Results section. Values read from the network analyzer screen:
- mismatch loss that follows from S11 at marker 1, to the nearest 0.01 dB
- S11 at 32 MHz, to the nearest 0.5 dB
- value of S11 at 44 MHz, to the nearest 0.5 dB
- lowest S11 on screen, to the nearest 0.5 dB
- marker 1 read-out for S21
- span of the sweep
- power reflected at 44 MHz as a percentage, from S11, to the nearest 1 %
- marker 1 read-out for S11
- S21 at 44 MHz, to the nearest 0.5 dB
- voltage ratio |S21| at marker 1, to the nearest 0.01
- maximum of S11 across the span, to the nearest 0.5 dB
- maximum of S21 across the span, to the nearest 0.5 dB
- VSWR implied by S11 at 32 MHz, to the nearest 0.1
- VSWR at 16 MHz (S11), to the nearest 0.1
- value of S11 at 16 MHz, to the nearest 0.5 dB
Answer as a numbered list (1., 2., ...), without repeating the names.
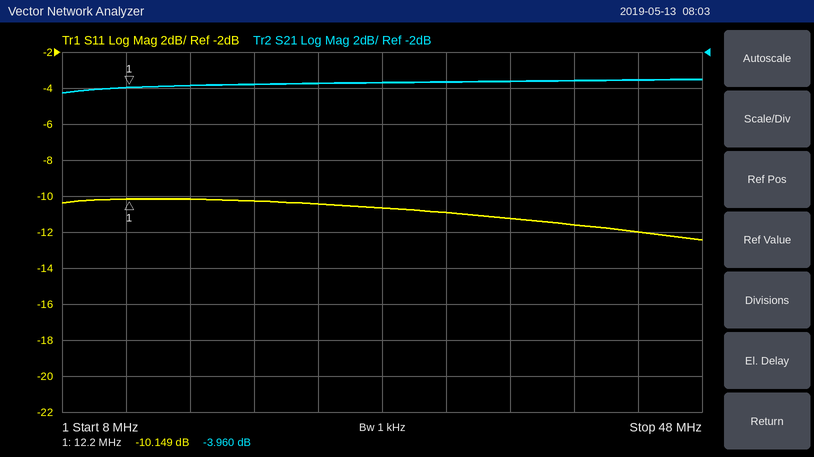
1. 0.44 dB
2. -11.0 dB
3. -12.0 dB
4. -12.5 dB
5. -3.960 dB
6. 40 MHz
7. 6 %
8. -10.149 dB
9. -3.5 dB
10. 0.63
11. -10.0 dB
12. -3.5 dB
13. 1.8
14. 1.9
15. -10.0 dB
